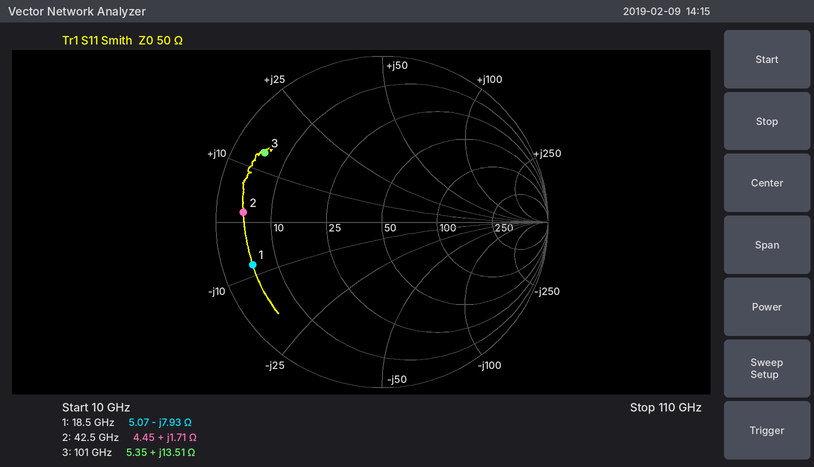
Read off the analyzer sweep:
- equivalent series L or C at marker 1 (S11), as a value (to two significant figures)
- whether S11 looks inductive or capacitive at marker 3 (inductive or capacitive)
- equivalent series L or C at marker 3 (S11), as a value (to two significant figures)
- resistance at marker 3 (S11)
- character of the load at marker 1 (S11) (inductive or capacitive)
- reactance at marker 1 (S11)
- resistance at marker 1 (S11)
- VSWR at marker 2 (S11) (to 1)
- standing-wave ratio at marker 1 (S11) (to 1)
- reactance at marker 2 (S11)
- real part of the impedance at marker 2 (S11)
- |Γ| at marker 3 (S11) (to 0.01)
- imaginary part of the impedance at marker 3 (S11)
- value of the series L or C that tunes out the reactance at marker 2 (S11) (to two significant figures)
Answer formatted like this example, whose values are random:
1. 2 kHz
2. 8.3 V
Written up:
1. 1.1 pF
2. inductive
3. 21 pH
4. 5.35 Ω
5. capacitive
6. -7.93 Ω
7. 5.07 Ω
8. 11
9. 10
10. +1.71 Ω
11. 4.45 Ω
12. 0.82
13. +13.51 Ω
14. 2.2 pF
